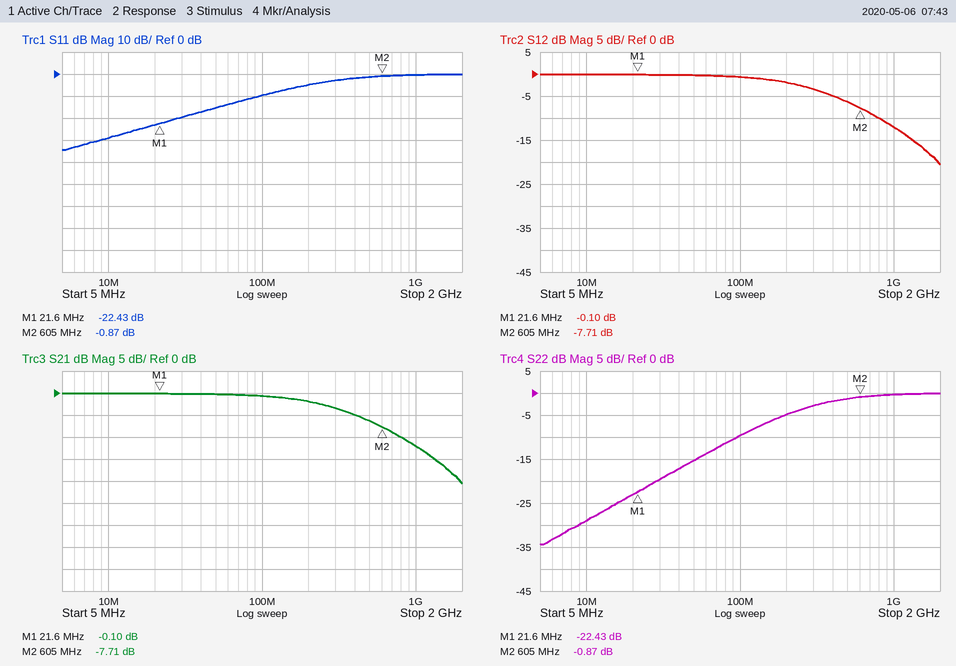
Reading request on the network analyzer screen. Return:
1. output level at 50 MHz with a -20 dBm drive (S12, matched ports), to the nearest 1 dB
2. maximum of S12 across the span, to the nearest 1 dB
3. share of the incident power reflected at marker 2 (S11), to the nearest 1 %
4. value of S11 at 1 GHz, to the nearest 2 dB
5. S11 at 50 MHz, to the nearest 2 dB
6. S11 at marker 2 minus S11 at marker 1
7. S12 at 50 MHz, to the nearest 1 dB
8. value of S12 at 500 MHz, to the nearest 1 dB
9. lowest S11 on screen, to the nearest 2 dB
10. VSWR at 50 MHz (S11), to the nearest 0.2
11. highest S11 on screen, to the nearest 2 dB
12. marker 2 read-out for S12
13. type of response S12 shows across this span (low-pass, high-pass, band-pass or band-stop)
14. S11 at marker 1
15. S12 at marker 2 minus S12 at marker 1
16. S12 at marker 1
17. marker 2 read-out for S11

-20 dBm
0 dB
82 %
0 dB
-16 dB
21.56 dB
0 dB
-6 dB
-34 dB
1.4
0 dB
-7.71 dB
low-pass
-22.43 dB
-7.61 dB
-0.10 dB
-0.87 dB
